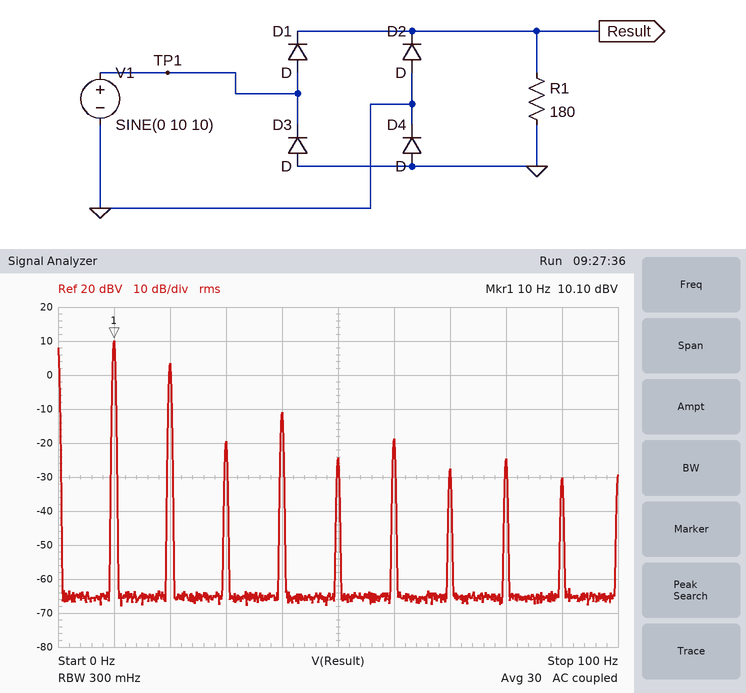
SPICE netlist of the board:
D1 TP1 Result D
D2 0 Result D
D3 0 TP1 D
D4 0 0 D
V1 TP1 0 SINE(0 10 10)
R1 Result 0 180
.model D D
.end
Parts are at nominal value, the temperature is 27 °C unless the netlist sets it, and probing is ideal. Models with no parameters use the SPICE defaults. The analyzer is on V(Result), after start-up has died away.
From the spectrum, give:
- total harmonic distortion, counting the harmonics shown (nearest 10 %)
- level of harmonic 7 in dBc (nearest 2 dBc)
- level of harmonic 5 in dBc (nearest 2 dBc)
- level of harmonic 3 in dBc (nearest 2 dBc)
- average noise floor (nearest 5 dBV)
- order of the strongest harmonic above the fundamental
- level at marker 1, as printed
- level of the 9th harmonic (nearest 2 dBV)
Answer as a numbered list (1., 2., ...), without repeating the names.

1. 50 %
2. -38 dBc
3. -34 dBc
4. -30 dBc
5. -65 dBV
6. 2
7. 10.10 dBV
8. -30 dBV
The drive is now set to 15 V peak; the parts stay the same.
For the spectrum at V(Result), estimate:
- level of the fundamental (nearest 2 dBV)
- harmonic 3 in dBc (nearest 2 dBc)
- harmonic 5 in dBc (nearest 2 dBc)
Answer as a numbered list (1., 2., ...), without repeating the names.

1. 14 dBV
2. -34 dBc
3. -38 dBc
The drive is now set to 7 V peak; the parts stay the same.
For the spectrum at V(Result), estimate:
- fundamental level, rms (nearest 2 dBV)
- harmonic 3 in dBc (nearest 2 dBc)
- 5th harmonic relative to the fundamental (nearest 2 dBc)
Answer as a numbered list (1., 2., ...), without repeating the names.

1. 6 dBV
2. -26 dBc
3. -32 dBc
